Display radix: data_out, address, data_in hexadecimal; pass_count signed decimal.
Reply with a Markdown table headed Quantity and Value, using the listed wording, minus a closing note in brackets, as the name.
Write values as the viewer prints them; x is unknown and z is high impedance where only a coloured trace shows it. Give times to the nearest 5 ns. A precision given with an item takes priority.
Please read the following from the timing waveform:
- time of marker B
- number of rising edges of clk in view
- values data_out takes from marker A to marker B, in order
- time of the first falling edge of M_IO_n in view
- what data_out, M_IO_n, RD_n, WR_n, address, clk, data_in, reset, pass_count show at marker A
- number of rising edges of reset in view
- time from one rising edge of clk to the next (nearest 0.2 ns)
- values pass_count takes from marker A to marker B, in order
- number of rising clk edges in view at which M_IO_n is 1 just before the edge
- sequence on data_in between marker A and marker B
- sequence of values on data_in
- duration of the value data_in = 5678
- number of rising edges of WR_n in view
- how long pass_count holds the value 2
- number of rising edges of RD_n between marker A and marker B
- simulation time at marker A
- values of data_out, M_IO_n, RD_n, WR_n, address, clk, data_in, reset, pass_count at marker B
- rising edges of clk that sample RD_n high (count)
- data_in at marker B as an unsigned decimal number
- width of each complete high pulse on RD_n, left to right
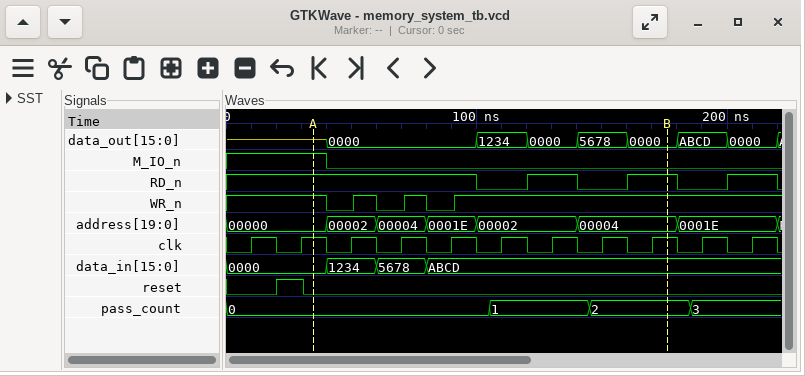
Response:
| Quantity | Value |
|---|---|
| time of marker B | 175 ns |
| number of rising edges of clk in view | 11 |
| values data_out takes from marker A to marker B, in order | z, 0000, 1234, 0000, 5678, 0000 |
| time of the first falling edge of M_IO_n in view | 40 ns |
| what data_out, M_IO_n, RD_n, WR_n, address, clk, data_in, reset, pass_count show at marker A | data_out=z, M_IO_n=1, RD_n=1, WR_n=1, address=00000, clk=1, data_in=0000, reset=0, pass_count=0 |
| number of rising edges of reset in view | 1 |
| time from one rising edge of clk to the next | 20 ns |
| values pass_count takes from marker A to marker B, in order | 0, 1, 2 |
| number of rising clk edges in view at which M_IO_n is 1 just before the edge | 2 |
| sequence on data_in between marker A and marker B | 0000, 1234, 5678, ABCD |
| sequence of values on data_in | 0000, 1234, 5678, ABCD |
| duration of the value data_in = 5678 | 20 ns |
| number of rising edges of WR_n in view | 3 |
| how long pass_count holds the value 2 | 40 ns |
| number of rising edges of RD_n between marker A and marker B | 2 |
| simulation time at marker A | 35 ns |
| values of data_out, M_IO_n, RD_n, WR_n, address, clk, data_in, reset, pass_count at marker B | data_out=0000, M_IO_n=0, RD_n=1, WR_n=1, address=00004, clk=1, data_in=ABCD, reset=0, pass_count=2 |
| rising edges of clk that sample RD_n high | 8 |
| data_in at marker B as an unsigned decimal number | 43981 |
| width of each complete high pulse on RD_n, left to right | 20 ns, 20 ns, 20 ns |
